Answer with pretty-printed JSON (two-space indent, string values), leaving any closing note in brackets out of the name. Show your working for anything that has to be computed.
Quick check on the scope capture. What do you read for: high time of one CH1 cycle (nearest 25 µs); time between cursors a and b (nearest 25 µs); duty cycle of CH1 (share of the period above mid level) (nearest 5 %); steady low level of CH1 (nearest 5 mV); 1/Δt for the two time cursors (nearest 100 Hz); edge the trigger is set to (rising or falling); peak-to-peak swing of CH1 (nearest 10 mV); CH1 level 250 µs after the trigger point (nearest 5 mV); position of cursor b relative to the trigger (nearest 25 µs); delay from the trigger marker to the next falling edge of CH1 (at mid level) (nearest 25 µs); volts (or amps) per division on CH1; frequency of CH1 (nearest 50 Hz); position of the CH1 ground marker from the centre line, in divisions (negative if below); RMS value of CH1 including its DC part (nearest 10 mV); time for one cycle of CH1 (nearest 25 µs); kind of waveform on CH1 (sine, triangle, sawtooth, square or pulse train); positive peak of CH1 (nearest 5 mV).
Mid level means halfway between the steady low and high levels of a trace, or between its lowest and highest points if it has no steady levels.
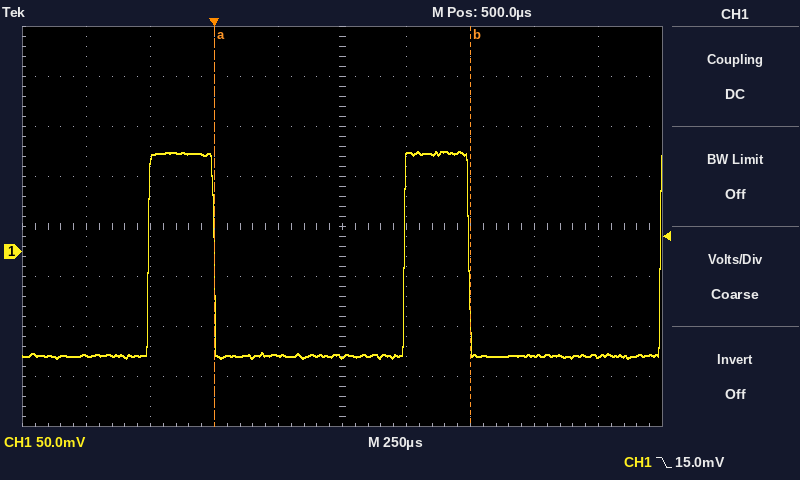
{
  "high time of one CH1 cycle": "250 µs",
  "time between cursors a and b": "1.000 ms",
  "duty cycle of CH1 (share of the period above mid level)": "250 µs / 1.000 ms ≈ 25 %",
  "steady low level of CH1": "-105 mV",
  "1/Δt for the two time cursors": "1 / 1.000 ms ≈ 1.0 kHz",
  "edge the trigger is set to": "falling",
  "peak-to-peak swing of CH1": "210 mV",
  "CH1 level 250 µs after the trigger point": "-105 mV",
  "position of cursor b relative to the trigger": "+1.000 ms",
  "delay from the trigger marker to the next falling edge of CH1 (at mid level)": "1.000 ms",
  "volts (or amps) per division on CH1": "50 mV",
  "frequency of CH1": "1 / 1.000 ms ≈ 1.00 kHz",
  "position of the CH1 ground marker from the centre line, in divisions": "-0.5 div",
  "RMS value of CH1 including its DC part": "√(0.25 × (100 mV)² + 0.75 × (-105 mV)²) ≈ 104 mV, so 100 mV to the nearest 10 mV",
  "time for one cycle of CH1": "1.000 ms",
  "kind of waveform on CH1": "pulse train",
  "positive peak of CH1": "100 mV"
}
